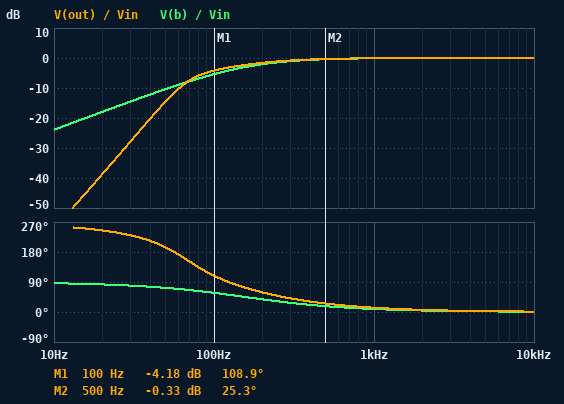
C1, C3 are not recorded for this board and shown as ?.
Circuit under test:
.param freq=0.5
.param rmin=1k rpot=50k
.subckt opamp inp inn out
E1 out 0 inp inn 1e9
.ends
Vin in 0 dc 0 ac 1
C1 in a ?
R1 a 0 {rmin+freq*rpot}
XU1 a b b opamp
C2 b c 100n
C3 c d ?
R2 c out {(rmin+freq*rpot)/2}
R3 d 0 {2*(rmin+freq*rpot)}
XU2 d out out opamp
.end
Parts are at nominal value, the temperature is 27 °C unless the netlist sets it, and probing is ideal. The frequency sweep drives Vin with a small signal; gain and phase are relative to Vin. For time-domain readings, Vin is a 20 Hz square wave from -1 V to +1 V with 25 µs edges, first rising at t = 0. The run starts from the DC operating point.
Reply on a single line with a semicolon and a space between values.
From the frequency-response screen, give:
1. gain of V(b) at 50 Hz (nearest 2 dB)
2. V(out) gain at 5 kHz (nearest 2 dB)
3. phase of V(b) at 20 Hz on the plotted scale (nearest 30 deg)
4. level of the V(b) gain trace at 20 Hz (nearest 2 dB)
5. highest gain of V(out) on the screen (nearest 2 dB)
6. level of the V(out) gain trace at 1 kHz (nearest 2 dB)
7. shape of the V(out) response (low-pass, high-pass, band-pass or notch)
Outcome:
-10 dB; 0 dB; 90 deg; -18 dB; 0 dB; 0 dB; high-pass
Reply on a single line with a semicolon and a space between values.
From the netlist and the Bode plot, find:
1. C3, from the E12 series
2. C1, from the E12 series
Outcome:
82 nF; 39 nF
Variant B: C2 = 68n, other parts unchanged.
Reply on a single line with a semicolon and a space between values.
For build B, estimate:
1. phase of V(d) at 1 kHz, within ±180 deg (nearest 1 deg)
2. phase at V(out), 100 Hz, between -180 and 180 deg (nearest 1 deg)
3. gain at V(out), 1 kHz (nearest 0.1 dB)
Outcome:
14 deg; 126 deg; -0.1 dB
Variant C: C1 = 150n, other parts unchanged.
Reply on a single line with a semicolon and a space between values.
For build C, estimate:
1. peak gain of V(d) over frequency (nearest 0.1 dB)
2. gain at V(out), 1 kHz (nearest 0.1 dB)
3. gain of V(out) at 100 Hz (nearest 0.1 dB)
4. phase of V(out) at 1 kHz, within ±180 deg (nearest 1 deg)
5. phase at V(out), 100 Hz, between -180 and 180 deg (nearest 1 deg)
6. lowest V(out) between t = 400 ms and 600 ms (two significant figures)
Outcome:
0.6 dB; 0 dB; 0.5 dB; 6 deg; 74 deg; -2.0 V
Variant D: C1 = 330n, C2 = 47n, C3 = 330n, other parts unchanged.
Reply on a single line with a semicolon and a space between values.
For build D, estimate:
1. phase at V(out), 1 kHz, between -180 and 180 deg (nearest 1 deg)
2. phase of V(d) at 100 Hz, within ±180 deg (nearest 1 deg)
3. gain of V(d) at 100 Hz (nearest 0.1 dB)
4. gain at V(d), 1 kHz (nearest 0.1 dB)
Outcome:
5 deg; 55 deg; -0.7 dB; 0 dB
